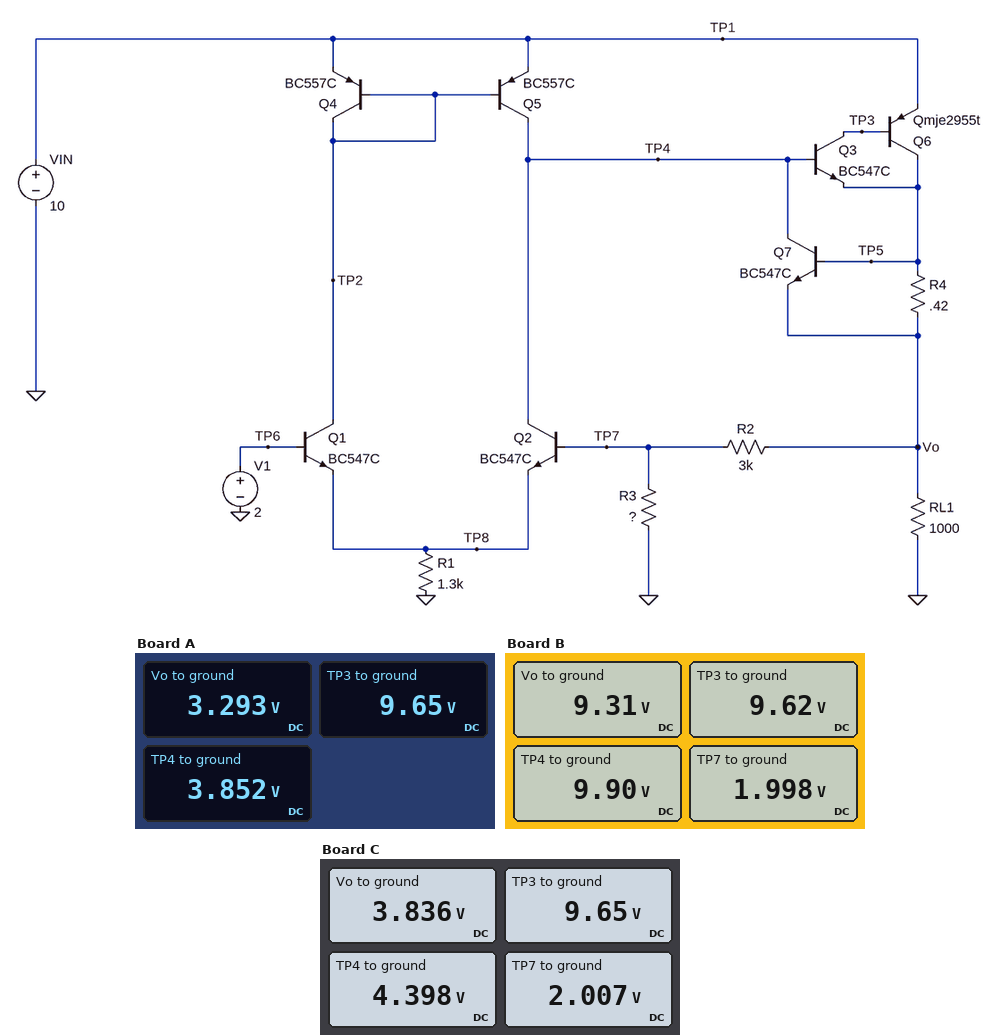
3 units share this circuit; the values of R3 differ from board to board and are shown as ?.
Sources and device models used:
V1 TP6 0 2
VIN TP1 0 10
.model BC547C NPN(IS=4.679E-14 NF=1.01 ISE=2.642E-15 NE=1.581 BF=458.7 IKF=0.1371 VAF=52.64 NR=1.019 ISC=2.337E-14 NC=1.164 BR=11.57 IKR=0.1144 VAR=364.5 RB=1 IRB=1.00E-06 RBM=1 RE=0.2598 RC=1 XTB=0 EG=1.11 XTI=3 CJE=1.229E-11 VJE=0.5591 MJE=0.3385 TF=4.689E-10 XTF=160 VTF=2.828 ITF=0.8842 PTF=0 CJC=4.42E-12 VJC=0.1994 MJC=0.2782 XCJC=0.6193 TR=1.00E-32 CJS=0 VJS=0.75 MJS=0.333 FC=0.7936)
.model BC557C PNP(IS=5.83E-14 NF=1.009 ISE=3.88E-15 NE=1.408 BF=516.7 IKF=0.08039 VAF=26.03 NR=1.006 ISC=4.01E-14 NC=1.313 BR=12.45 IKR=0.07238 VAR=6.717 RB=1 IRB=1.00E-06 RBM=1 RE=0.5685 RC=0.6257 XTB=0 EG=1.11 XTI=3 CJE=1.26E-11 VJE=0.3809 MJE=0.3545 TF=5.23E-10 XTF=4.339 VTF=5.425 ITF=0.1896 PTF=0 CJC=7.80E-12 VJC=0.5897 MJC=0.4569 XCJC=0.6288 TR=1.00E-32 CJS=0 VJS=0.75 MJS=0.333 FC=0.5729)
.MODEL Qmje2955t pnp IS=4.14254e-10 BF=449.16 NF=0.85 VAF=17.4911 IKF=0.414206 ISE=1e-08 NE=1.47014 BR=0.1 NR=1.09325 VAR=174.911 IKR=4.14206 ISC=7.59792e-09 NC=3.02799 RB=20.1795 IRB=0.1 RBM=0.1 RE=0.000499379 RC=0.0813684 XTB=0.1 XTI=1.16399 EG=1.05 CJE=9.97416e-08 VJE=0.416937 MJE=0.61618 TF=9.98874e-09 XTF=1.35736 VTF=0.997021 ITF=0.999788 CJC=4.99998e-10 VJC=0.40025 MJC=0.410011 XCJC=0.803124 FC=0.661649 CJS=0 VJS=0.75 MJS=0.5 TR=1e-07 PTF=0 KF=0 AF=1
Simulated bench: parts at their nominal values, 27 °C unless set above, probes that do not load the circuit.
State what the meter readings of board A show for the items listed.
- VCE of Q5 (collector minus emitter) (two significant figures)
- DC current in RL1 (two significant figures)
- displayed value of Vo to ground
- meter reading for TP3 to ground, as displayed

-6.1 V
3.3 mA
3.293 V
9.65 V
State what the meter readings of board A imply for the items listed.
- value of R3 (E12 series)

4.7 kΩ
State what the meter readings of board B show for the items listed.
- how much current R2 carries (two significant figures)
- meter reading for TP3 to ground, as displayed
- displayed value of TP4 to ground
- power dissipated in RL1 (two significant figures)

2.4 mA
9.62 V
9.90 V
87 mW
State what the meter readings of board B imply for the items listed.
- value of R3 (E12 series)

820 Ω
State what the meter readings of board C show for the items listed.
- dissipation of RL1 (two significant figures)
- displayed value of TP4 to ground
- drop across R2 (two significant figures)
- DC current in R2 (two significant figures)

15 mW
4.398 V
1.8 V
610 µA
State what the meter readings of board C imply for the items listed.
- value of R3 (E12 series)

3.3 kΩ
